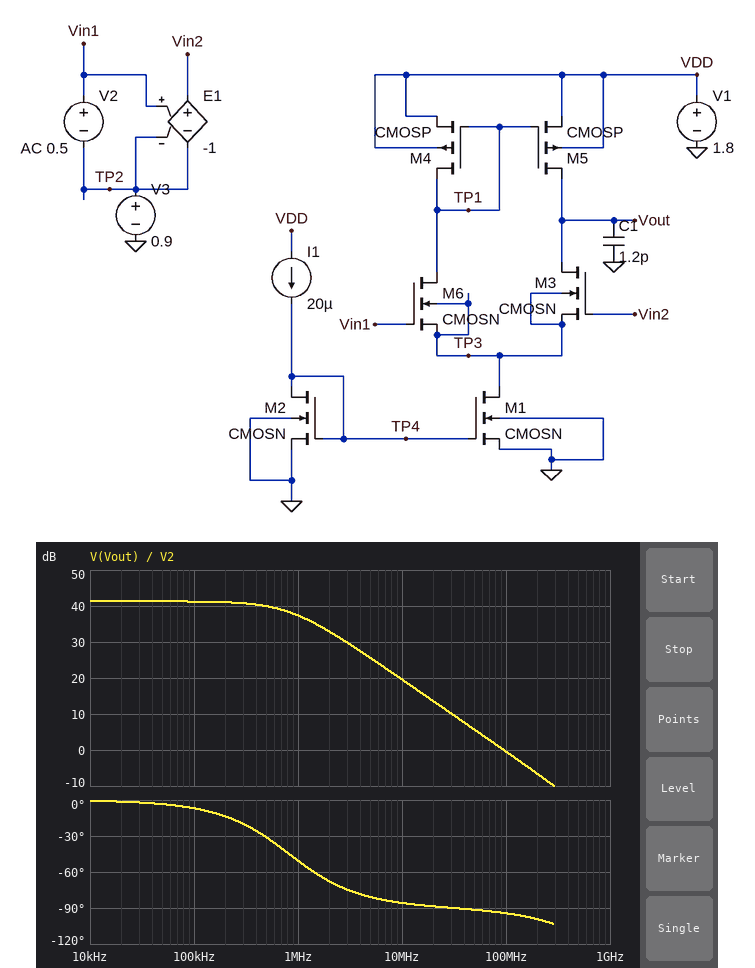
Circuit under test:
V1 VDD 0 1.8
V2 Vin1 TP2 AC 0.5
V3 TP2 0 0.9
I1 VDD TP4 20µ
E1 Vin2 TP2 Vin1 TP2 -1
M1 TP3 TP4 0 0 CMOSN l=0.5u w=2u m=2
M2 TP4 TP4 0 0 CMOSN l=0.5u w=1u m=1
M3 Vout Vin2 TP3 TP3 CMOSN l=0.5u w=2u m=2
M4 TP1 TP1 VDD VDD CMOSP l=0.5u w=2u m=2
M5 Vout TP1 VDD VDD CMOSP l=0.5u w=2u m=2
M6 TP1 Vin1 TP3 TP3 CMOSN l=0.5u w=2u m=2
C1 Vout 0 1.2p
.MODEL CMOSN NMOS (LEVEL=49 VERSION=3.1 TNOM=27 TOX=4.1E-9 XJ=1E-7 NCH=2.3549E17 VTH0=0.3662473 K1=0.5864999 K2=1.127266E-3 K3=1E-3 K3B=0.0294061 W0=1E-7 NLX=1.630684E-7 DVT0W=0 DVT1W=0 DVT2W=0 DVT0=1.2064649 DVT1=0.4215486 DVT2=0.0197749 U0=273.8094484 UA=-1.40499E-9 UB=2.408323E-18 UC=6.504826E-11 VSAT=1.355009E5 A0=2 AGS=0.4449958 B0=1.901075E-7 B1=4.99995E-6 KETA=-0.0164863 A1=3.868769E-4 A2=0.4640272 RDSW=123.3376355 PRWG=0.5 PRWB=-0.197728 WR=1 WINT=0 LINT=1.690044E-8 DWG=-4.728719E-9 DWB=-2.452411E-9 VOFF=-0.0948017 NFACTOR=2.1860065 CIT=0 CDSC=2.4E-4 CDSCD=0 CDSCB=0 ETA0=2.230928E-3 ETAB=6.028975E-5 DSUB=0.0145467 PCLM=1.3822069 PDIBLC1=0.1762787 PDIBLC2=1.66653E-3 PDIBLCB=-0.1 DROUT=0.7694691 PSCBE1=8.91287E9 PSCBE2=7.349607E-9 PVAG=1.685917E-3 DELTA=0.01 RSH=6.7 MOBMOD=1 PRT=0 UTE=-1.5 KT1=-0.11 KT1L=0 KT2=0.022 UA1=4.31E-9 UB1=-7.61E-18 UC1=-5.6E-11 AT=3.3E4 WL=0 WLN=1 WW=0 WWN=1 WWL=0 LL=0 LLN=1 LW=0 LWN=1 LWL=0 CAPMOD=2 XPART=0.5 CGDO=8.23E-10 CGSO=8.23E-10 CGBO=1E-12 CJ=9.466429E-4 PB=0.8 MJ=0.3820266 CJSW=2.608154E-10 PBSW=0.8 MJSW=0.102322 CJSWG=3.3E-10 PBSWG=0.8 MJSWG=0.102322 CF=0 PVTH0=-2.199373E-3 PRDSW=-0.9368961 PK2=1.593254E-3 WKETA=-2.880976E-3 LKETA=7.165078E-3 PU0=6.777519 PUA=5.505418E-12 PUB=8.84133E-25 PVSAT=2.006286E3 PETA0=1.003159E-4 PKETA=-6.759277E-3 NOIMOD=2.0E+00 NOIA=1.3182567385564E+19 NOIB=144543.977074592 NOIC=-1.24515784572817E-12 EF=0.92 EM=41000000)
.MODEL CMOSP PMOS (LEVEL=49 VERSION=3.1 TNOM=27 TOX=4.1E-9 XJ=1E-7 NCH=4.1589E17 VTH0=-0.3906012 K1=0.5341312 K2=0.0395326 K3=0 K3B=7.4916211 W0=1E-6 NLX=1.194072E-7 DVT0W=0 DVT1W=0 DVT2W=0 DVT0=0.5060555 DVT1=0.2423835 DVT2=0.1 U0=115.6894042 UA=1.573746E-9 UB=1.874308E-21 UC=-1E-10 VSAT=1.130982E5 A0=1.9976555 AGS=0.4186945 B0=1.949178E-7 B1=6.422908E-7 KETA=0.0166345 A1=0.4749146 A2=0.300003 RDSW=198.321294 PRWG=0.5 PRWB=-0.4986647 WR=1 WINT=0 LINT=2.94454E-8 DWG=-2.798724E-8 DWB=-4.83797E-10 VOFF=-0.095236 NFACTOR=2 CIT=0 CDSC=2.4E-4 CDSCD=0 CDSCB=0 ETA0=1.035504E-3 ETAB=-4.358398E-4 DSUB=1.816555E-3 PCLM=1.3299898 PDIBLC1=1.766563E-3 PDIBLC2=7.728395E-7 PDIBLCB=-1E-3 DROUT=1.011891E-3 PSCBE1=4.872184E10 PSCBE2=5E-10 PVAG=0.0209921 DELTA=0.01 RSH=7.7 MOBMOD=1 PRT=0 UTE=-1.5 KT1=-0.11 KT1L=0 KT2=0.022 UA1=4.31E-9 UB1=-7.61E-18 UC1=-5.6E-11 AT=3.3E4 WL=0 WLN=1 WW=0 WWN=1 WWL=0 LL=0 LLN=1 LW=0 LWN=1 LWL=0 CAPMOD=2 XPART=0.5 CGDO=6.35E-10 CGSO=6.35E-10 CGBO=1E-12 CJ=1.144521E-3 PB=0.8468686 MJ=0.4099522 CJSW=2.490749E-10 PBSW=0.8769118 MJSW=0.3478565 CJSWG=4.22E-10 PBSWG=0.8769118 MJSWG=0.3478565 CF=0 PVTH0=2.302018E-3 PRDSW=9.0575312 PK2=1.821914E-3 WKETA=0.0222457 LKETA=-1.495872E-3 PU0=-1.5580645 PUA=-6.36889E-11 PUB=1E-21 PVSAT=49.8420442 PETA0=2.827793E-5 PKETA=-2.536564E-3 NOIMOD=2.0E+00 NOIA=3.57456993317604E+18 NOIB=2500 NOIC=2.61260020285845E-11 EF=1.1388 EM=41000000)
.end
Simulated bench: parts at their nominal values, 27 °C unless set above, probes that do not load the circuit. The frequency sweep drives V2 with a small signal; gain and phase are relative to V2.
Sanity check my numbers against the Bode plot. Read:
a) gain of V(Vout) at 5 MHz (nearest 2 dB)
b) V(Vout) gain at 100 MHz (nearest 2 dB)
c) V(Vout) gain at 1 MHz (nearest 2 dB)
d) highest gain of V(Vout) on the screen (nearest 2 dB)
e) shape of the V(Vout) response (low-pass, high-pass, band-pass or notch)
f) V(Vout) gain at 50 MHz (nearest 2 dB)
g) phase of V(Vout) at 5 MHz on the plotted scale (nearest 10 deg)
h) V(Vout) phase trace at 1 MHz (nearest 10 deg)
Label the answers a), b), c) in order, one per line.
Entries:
a) 26 dB
b) 0 dB
c) 38 dB
d) 42 dB
e) low-pass
f) 6 dB
g) -80 deg
h) -50 deg
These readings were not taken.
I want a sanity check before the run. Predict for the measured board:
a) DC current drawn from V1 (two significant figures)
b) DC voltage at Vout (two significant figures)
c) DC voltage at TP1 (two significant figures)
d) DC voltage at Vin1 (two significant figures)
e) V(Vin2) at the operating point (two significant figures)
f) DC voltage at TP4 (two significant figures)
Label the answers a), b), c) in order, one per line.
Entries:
a) 91 µA
b) 980 mV
c) 980 mV
d) 900 mV
e) 900 mV
f) 720 mV
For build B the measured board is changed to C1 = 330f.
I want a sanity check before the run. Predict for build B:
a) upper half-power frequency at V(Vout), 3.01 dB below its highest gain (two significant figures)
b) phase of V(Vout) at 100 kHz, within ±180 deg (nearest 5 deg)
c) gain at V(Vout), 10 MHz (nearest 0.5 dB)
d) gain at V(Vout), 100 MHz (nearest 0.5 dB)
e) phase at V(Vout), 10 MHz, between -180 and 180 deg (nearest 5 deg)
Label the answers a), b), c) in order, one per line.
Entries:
a) 2.9 MHz
b) 0 deg
c) 30.5 dB
d) 10.5 dB
e) -75 deg
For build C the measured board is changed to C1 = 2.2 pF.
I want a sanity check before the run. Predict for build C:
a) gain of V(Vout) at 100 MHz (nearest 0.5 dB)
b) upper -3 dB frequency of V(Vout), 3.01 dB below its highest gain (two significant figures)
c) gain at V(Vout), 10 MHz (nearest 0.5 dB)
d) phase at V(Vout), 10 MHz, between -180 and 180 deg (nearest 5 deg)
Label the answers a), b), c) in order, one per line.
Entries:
a) -5.5 dB
b) 450 kHz
c) 14.5 dB
d) -90 deg
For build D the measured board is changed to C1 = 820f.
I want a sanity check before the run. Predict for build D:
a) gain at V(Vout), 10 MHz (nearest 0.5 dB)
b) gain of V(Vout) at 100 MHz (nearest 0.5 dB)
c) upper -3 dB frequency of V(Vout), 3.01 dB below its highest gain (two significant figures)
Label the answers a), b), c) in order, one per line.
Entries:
a) 23.0 dB
b) 3.0 dB
c) 1.2 MHz
